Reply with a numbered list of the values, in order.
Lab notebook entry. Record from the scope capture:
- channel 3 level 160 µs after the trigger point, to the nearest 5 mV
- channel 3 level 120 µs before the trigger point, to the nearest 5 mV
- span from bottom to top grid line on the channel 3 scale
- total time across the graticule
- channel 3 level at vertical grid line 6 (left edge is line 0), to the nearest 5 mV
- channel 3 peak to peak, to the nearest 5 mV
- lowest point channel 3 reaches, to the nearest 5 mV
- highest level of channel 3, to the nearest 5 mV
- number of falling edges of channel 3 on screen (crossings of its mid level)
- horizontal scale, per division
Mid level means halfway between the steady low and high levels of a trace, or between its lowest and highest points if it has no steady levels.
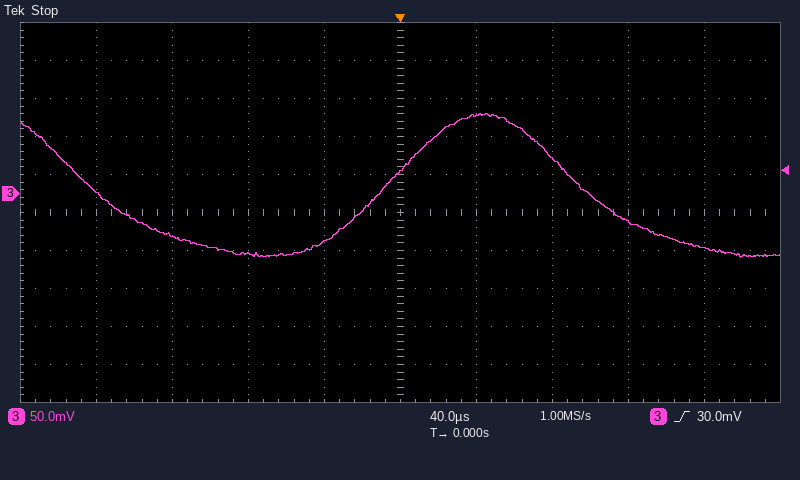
1. -70 mV
2. -55 mV
3. 500 mV
4. 400 µs
5. 105 mV
6. 190 mV
7. -85 mV
8. 105 mV
9. 2
10. 40 µs
